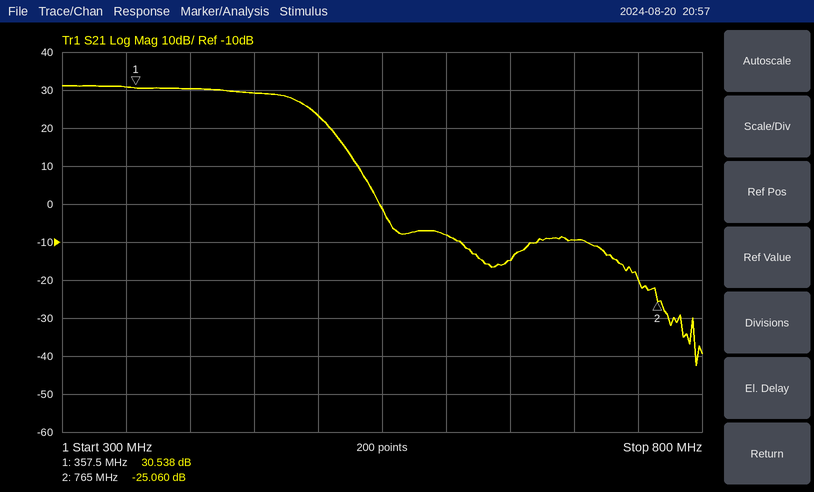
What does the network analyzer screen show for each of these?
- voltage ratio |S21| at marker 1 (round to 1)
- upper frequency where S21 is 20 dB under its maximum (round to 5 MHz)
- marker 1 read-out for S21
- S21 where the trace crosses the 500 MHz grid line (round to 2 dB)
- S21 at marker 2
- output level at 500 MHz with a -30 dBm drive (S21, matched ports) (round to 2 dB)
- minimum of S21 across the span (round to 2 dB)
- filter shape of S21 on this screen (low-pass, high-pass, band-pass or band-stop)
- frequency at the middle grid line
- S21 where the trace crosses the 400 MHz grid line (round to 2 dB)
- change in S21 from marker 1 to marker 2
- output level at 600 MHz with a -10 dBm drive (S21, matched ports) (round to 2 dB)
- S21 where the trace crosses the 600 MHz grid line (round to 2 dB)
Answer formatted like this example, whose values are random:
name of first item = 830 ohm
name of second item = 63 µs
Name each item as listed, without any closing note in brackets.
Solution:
voltage ratio |S21| at marker 1 = 34
upper frequency where S21 is 20 dB under its maximum = 530 MHz
marker 1 read-out for S21 = 30.538 dB
S21 where the trace crosses the 500 MHz grid line = 24 dB
S21 at marker 2 = -25.060 dB
output level at 500 MHz with a -30 dBm drive (S21, matched ports) = -6 dBm
minimum of S21 across the span = -42 dB
filter shape of S21 on this screen = low-pass
frequency at the middle grid line = 550 MHz
S21 where the trace crosses the 400 MHz grid line = 30 dB
change in S21 from marker 1 to marker 2 = -55.598 dB
output level at 600 MHz with a -10 dBm drive (S21, matched ports) = -18 dBm
S21 where the trace crosses the 600 MHz grid line = -8 dB
